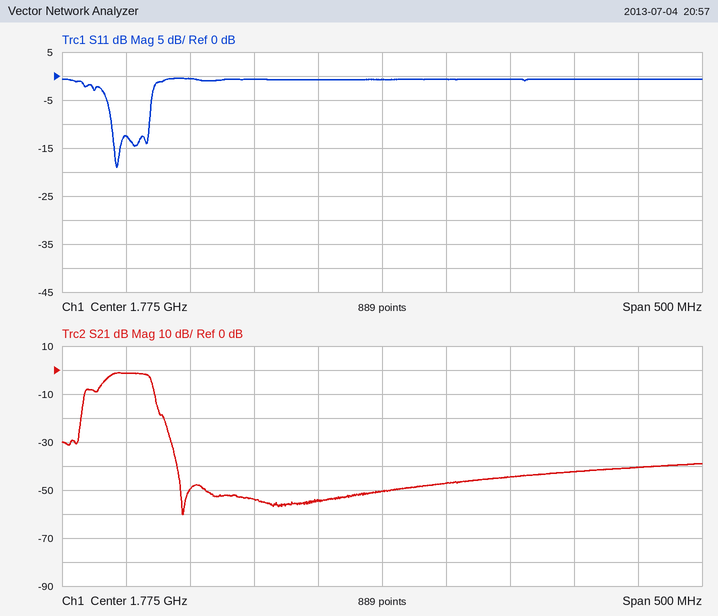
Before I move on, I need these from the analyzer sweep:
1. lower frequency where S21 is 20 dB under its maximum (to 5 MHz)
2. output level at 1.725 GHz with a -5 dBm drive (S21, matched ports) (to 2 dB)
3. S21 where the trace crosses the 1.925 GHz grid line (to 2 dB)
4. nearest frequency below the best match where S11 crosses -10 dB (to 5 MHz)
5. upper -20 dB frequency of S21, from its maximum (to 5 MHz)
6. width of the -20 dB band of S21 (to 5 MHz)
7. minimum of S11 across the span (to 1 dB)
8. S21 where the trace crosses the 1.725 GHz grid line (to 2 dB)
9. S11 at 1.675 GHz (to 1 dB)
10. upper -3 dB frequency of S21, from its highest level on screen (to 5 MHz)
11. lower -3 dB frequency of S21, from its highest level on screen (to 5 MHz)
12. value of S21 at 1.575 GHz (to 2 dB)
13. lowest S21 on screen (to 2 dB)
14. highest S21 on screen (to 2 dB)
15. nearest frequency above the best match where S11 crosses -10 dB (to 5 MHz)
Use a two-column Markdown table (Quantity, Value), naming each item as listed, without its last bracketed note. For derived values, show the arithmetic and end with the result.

| Quantity | Value |
|---|---|
| lower frequency where S21 is 20 dB under its maximum | 1.540 GHz |
| output level at 1.725 GHz with a -5 dBm drive (S21, matched ports) | -5 dBm + (-54 dB) = -60 dBm |
| S21 where the trace crosses the 1.925 GHz grid line | -42 dB |
| nearest frequency below the best match where S11 crosses -10 dB | 1.565 GHz |
| upper -20 dB frequency of S21, from its maximum | 1.605 GHz |
| width of the -20 dB band of S21 | 1.605 GHz − 1.540 GHz = 65 MHz |
| minimum of S11 across the span | -19 dB |
| S21 where the trace crosses the 1.725 GHz grid line | -54 dB |
| S11 at 1.675 GHz | -1 dB |
| upper -3 dB frequency of S21, from its highest level on screen | 1.595 GHz |
| lower -3 dB frequency of S21, from its highest level on screen | 1.560 GHz |
| value of S21 at 1.575 GHz | -2 dB |
| lowest S21 on screen | -60 dB |
| highest S21 on screen | -2 dB |
| nearest frequency above the best match where S11 crosses -10 dB | 1.595 GHz |
